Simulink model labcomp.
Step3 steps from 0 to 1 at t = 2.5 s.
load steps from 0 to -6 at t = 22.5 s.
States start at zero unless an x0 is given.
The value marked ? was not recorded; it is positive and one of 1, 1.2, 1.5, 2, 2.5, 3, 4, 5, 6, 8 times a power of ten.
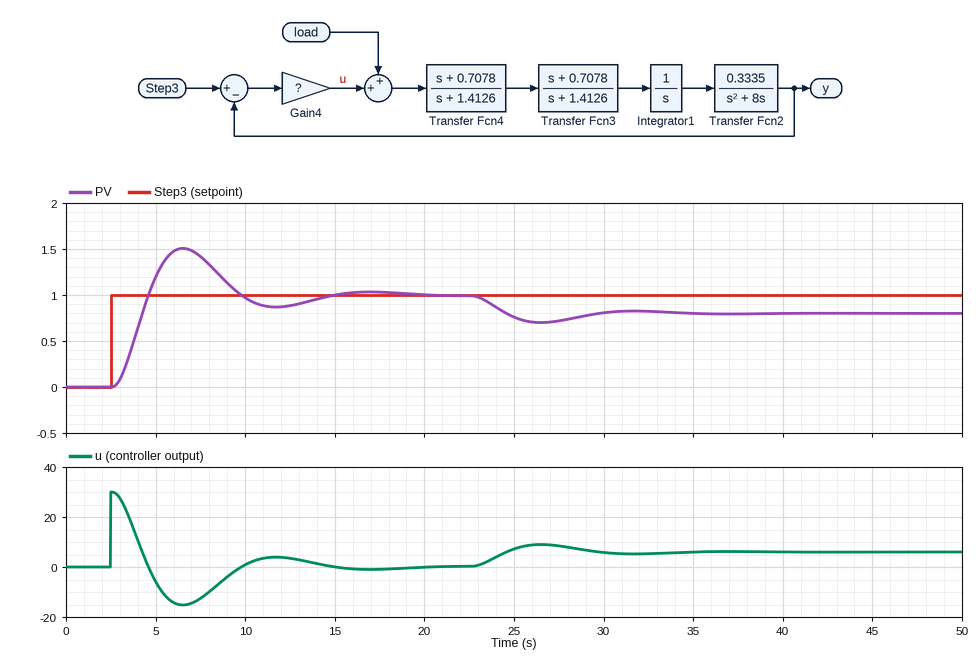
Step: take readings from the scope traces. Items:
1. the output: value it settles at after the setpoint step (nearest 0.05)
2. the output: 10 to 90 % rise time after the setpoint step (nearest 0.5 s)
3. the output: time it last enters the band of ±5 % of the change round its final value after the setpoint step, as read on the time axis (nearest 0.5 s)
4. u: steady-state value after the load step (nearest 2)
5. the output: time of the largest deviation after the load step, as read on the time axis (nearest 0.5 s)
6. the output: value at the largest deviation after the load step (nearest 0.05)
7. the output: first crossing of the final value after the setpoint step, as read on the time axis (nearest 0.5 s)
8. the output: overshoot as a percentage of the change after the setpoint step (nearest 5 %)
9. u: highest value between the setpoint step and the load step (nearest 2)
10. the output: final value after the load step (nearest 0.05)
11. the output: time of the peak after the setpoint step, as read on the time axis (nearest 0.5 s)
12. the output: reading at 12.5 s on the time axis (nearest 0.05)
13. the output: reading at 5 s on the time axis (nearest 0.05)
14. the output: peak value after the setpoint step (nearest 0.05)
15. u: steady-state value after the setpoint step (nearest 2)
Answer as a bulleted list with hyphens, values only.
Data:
- 1.00
- 1.5 s
- 14.0 s
- 6
- 26.5 s
- 0.70
- 4.5 s
- 50 %
- 30
- 0.80
- 6.5 s
- 0.90
- 1.20
- 1.50
- 0
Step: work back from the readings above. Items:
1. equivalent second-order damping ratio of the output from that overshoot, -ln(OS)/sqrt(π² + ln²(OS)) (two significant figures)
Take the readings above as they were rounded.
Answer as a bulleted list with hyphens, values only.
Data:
- 0.22
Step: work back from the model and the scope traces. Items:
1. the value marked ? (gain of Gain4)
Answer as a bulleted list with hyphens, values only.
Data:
- 30
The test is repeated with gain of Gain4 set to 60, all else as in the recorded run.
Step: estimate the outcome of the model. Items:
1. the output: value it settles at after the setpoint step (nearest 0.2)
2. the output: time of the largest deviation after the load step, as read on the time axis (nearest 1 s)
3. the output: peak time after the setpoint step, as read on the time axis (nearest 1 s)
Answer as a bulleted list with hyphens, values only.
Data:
- 1.0
- 25 s
- 5 s
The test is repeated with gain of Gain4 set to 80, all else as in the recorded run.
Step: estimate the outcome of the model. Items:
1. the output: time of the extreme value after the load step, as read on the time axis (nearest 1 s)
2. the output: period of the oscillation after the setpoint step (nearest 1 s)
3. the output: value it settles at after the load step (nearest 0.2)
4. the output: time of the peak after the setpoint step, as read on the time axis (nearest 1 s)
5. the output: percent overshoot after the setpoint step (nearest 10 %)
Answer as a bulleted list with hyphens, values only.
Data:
- 25 s
- 4 s
- 1.0
- 5 s
- 60 %
